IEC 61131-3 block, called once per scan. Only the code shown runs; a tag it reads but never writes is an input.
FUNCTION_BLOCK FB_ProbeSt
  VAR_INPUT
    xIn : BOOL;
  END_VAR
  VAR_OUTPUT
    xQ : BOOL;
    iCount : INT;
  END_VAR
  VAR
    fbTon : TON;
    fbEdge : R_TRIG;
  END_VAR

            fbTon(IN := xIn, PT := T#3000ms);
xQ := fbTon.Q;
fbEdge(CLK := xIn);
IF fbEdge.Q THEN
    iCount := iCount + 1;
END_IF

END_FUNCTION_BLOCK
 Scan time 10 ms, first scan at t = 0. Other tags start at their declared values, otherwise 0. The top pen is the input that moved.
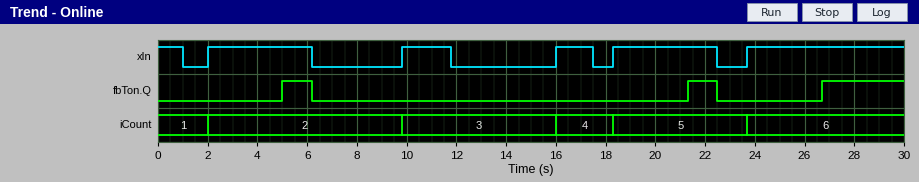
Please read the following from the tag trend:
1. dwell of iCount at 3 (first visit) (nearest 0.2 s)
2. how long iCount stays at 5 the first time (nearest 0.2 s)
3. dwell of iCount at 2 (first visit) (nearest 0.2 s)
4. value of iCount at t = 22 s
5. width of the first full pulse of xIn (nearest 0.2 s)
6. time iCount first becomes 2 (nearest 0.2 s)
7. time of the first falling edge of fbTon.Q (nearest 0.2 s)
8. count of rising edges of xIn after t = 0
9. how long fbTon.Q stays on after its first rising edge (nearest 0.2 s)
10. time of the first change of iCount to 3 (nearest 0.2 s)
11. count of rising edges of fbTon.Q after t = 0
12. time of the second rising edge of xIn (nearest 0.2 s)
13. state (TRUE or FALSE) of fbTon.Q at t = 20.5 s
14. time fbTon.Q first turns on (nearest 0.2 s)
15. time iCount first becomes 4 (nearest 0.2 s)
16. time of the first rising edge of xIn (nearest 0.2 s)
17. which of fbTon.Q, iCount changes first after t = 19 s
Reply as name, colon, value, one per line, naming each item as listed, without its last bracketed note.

dwell of iCount at 3 (first visit): 6.2 s
how long iCount stays at 5 the first time: 5.4 s
dwell of iCount at 2 (first visit): 7.8 s
value of iCount at t = 22 s: 5
width of the first full pulse of xIn: 4.2 s
time iCount first becomes 2: 2.0 s
time of the first falling edge of fbTon.Q: 6.2 s
count of rising edges of xIn after t = 0: 5
how long fbTon.Q stays on after its first rising edge: 1.2 s
time of the first change of iCount to 3: 9.8 s
count of rising edges of fbTon.Q after t = 0: 3
time of the second rising edge of xIn: 9.8 s
state (TRUE or FALSE) of fbTon.Q at t = 20.5 s: FALSE
time fbTon.Q first turns on: 5.0 s
time iCount first becomes 4: 16.0 s
time of the first rising edge of xIn: 2.0 s
which of fbTon.Q, iCount changes first after t = 19 s: fbTon.Q
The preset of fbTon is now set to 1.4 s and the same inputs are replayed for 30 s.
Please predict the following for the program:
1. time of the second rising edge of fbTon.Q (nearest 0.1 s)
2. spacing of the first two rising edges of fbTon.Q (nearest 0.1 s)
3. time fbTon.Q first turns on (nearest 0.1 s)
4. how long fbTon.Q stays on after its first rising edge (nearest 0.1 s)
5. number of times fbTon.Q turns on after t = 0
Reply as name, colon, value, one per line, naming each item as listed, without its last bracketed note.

time of the second rising edge of fbTon.Q: 11.2 s
spacing of the first two rising edges of fbTon.Q: 7.8 s
time fbTon.Q first turns on: 3.4 s
how long fbTon.Q stays on after its first rising edge: 2.8 s
number of times fbTon.Q turns on after t = 0: 5
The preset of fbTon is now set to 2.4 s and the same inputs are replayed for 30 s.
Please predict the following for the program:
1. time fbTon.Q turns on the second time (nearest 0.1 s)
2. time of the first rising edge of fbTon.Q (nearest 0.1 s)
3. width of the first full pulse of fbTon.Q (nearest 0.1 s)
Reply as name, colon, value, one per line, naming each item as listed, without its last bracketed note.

time fbTon.Q turns on the second time: 20.7 s
time of the first rising edge of fbTon.Q: 4.4 s
width of the first full pulse of fbTon.Q: 1.8 s
